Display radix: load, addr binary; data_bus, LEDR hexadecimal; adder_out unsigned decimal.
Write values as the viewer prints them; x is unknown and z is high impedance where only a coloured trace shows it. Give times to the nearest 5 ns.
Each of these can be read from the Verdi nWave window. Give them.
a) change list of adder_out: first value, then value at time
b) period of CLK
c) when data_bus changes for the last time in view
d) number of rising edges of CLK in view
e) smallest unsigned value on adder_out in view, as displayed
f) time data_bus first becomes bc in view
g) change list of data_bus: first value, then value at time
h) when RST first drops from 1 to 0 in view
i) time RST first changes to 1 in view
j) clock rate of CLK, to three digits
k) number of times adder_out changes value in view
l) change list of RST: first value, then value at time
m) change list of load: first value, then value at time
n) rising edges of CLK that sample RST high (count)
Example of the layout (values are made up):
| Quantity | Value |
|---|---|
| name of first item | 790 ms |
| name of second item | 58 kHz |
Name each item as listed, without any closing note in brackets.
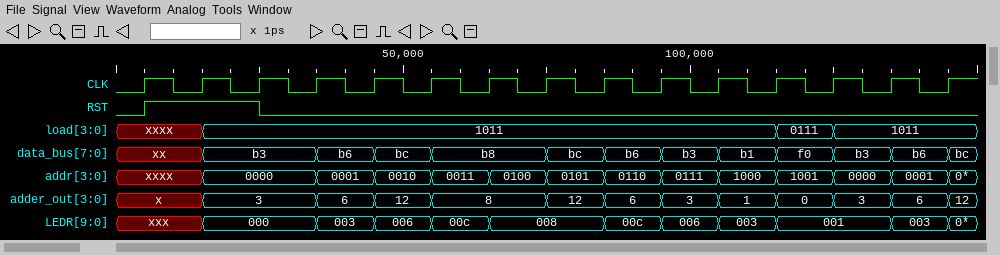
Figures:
| Quantity | Value |
|---|---|
| change list of adder_out: first value, then value at time | x, 3 at 15 ns, 6 at 35 ns, 12 at 45 ns, 8 at 55 ns, 12 at 75 ns, 6 at 85 ns, 3 at 95 ns, 1 at 105 ns, 0 at 115 ns, 3 at 125 ns, 6 at 135 ns, 12 at 145 ns |
| period of CLK | 10 ns |
| when data_bus changes for the last time in view | 145 ns |
| number of rising edges of CLK in view | 15 |
| smallest unsigned value on adder_out in view, as displayed | 0 |
| time data_bus first becomes bc in view | 45 ns |
| change list of data_bus: first value, then value at time | xx, b3 at 15 ns, b6 at 35 ns, bc at 45 ns, b8 at 55 ns, bc at 75 ns, b6 at 85 ns, b3 at 95 ns, b1 at 105 ns, f0 at 115 ns, b3 at 125 ns, b6 at 135 ns, bc at 145 ns |
| when RST first drops from 1 to 0 in view | 25 ns |
| time RST first changes to 1 in view | 5 ns |
| clock rate of CLK, to three digits | 100 MHz |
| number of times adder_out changes value in view | 12 |
| change list of RST: first value, then value at time | 0, 1 at 5 ns, 0 at 25 ns |
| change list of load: first value, then value at time | xxxx, 1011 at 15 ns, 0111 at 115 ns, 1011 at 125 ns |
| rising edges of CLK that sample RST high | 2 |
